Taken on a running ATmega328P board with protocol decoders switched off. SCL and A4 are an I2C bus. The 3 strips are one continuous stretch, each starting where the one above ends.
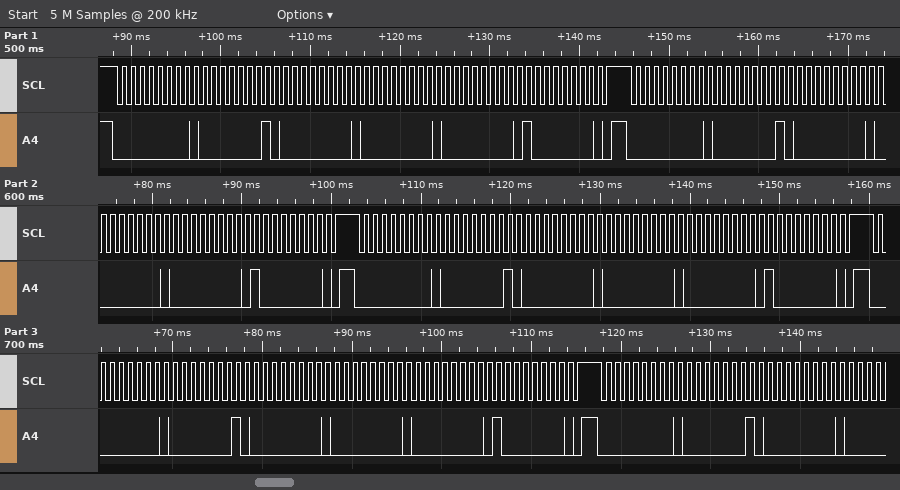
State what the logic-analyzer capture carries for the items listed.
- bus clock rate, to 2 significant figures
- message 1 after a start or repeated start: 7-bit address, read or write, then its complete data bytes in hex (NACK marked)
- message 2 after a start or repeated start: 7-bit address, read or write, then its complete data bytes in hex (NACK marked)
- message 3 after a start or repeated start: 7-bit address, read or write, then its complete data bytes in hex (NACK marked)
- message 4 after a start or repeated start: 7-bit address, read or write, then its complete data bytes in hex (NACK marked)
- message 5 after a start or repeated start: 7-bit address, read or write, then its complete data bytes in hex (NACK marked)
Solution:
1000 Hz
0x00 write: 01 00 00 00 80
0x00 write: 01 00 00 00 80
0x00 write: 01 00 00 00 80
0x00 write: 01 00 00 00 80
0x00 write: 01 00
